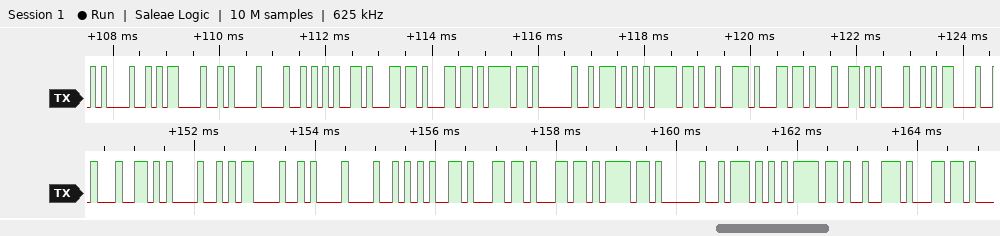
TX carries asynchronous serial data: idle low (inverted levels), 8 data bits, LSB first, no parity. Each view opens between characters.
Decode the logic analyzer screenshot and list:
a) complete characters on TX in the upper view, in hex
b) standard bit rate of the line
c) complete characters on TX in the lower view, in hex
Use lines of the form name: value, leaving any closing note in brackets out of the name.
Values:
complete characters on TX in the upper view, in hex: BD, E5, EB, 6F, 35, 27, 27, 21, BF, 51, 21, 1B, 27, 37, BD, E5
standard bit rate of the line: 9600 baud
complete characters on TX in the lower view, in hex: 37, BD, E5, EB, 6F, 35, 27, 27, 21, BF, 51, 21, 1B, 27
